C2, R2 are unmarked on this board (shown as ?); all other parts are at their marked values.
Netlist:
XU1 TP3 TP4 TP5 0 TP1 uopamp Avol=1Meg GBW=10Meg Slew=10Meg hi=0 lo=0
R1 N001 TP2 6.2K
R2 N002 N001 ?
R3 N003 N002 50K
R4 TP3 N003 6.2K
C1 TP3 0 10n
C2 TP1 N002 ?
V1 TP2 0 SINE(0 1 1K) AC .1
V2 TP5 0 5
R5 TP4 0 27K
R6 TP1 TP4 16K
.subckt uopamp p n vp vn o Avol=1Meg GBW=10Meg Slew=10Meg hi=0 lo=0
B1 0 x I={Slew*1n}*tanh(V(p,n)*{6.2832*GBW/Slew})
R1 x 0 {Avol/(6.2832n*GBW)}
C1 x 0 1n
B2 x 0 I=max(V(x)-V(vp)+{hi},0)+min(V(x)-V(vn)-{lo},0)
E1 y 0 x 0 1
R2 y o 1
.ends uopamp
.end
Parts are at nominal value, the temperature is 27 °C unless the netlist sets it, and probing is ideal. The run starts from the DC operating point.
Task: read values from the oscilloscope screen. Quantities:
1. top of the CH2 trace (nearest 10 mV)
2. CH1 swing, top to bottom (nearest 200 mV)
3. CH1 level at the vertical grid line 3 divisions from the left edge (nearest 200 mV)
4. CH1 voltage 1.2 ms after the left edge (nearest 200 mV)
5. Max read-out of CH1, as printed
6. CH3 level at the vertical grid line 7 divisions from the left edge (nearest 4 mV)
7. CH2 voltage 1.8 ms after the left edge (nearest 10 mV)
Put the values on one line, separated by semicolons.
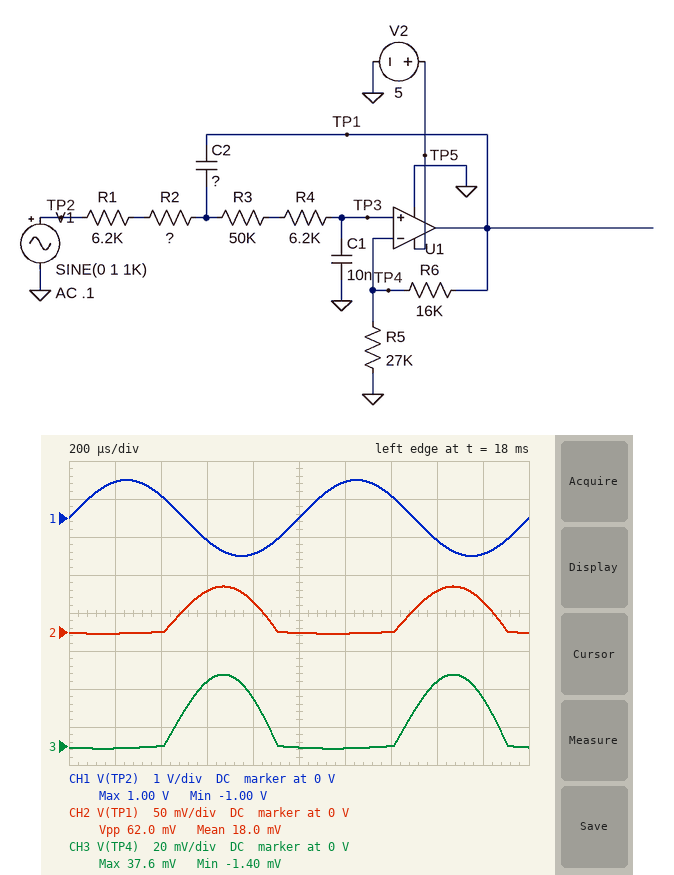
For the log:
60 mV; 2.0 V; -600 mV; 1.0 V; 1.00 V; 0 V; 40 mV
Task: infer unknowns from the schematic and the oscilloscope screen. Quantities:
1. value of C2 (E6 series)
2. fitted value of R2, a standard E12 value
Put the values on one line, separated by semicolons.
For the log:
6.8 nF; 150 kΩ
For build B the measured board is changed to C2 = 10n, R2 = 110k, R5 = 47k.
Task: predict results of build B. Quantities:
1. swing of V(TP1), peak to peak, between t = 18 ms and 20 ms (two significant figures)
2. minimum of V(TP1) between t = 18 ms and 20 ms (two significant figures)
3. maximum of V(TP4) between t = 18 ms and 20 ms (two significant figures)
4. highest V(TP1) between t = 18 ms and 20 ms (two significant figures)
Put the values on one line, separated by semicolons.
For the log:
50 mV; -2.1 mV; 36 mV; 48 mV
